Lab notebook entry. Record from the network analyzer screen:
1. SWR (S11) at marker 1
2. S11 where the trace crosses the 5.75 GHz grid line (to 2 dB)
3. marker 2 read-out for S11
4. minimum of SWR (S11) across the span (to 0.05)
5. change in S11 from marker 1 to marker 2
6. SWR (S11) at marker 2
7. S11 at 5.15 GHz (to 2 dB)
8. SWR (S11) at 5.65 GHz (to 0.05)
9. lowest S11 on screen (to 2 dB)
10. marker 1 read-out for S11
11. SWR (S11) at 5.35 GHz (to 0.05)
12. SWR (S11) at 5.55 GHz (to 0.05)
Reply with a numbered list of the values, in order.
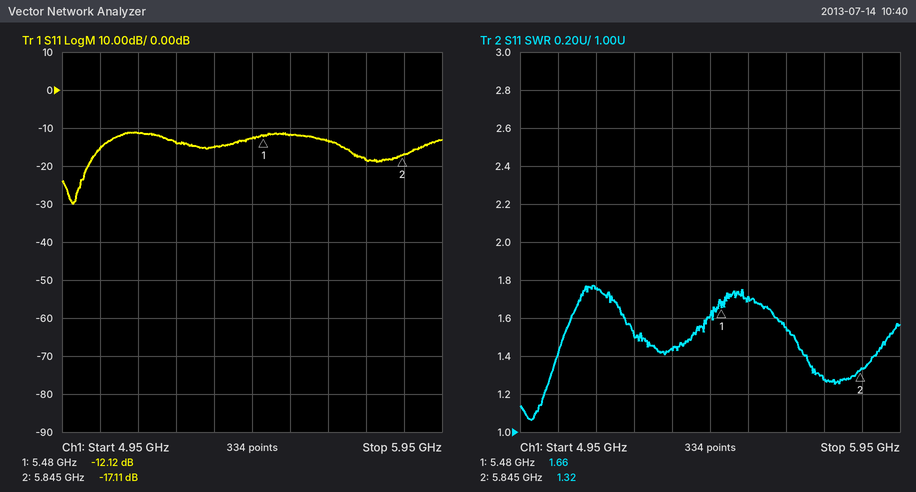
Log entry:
1. 1.66
2. -18 dB
3. -17.11 dB
4. 1.05
5. -4.99 dB
6. 1.32
7. -12 dB
8. 1.55
9. -30 dB
10. -12.12 dB
11. 1.45
12. 1.70
